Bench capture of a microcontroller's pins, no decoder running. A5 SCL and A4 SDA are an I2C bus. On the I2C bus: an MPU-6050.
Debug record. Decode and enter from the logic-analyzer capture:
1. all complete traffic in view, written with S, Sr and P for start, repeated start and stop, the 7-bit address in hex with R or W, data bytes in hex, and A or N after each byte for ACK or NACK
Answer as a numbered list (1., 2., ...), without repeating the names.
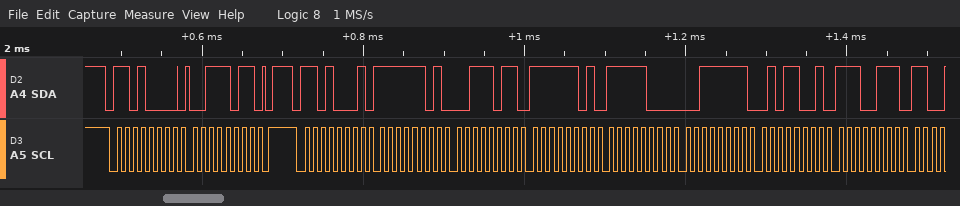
1. S 68W A 3B A P S 68R A FD A 3B A FD A F8 A 3F A 59 A E7 A
